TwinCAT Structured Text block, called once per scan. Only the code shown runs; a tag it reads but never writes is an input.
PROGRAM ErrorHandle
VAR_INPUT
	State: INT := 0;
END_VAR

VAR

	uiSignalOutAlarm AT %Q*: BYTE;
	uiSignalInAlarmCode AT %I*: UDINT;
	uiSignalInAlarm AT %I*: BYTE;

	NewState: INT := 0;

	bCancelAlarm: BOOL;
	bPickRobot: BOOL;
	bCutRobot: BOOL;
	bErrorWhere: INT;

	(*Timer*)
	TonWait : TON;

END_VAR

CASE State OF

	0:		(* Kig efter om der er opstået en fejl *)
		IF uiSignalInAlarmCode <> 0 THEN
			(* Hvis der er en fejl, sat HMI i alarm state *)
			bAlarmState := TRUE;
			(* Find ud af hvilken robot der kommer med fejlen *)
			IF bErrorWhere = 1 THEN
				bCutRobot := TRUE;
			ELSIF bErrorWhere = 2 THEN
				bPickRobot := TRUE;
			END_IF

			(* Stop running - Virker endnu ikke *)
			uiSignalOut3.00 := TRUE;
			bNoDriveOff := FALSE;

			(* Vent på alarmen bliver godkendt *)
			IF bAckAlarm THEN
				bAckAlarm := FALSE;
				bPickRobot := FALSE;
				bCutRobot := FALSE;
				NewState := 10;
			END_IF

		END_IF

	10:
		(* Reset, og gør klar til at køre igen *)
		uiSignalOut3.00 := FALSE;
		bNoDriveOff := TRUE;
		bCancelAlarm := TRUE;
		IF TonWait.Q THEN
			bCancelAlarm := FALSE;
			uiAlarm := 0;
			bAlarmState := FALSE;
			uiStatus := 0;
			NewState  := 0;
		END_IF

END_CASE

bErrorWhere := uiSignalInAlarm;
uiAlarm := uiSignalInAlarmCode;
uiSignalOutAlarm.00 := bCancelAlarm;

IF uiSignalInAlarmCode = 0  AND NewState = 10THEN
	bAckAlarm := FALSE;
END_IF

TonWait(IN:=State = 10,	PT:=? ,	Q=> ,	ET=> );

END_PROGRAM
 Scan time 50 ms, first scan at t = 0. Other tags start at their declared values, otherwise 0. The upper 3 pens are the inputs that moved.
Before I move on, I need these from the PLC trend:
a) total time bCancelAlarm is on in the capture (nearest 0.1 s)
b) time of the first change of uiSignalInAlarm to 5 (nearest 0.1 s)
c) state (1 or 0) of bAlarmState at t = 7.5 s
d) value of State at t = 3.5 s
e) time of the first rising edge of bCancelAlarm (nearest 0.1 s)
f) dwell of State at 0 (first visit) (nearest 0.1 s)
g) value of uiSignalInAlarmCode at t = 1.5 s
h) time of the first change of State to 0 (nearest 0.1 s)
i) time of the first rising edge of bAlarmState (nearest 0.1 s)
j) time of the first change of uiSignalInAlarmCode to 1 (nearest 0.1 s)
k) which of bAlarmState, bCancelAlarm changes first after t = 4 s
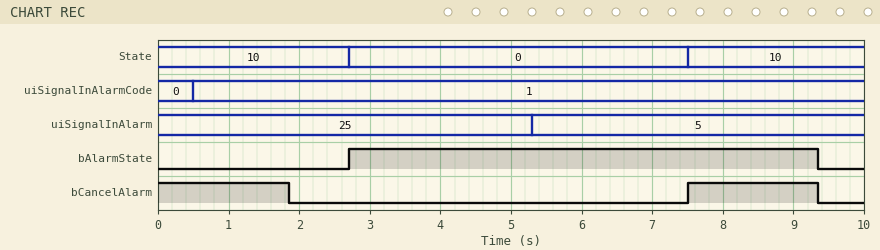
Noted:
3.7 s
5.3 s
1
0
7.5 s
4.8 s
1
2.7 s
2.7 s
0.5 s
bCancelAlarm
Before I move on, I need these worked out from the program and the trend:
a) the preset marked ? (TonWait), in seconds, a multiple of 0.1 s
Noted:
1.8 s
